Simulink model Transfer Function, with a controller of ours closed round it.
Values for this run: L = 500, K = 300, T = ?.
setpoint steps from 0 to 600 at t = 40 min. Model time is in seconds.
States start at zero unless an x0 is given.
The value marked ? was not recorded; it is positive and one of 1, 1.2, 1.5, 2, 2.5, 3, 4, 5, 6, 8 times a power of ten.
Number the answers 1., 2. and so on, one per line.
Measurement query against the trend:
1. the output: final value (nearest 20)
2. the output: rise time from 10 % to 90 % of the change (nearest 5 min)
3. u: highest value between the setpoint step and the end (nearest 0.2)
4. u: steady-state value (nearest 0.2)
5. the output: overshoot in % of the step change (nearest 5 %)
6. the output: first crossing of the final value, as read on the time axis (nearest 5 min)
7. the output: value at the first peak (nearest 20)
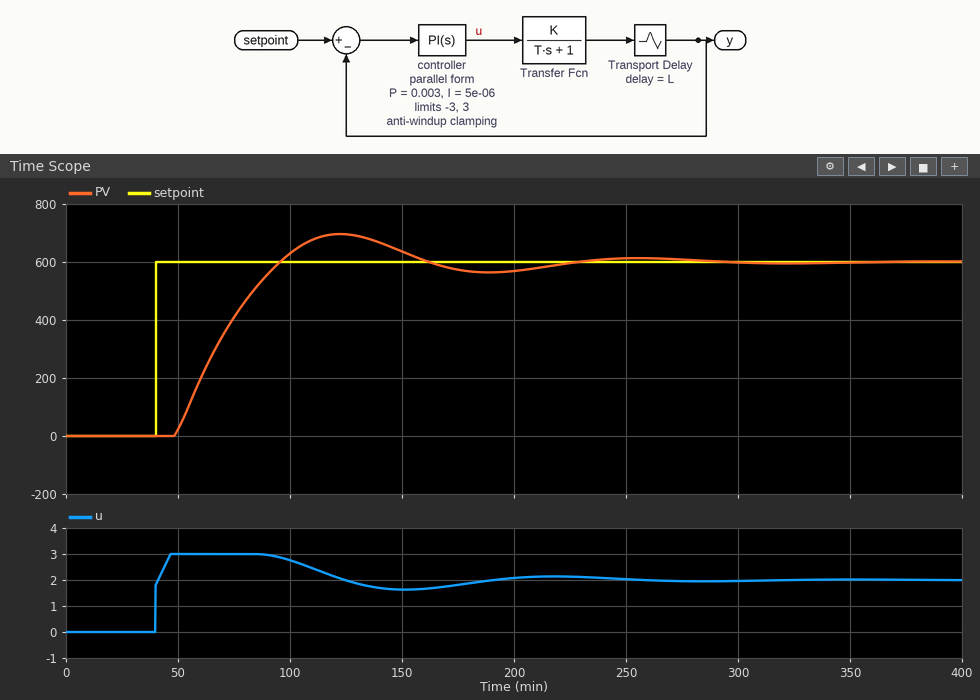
1. 600
2. 35 min
3. 3.0
4. 2.0
5. 15 %
6. 95 min
7. 700
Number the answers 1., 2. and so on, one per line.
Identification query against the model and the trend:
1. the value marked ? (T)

1. 2500
